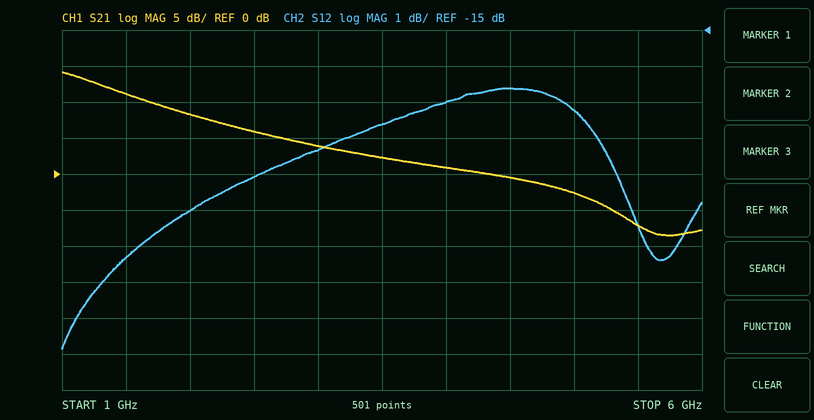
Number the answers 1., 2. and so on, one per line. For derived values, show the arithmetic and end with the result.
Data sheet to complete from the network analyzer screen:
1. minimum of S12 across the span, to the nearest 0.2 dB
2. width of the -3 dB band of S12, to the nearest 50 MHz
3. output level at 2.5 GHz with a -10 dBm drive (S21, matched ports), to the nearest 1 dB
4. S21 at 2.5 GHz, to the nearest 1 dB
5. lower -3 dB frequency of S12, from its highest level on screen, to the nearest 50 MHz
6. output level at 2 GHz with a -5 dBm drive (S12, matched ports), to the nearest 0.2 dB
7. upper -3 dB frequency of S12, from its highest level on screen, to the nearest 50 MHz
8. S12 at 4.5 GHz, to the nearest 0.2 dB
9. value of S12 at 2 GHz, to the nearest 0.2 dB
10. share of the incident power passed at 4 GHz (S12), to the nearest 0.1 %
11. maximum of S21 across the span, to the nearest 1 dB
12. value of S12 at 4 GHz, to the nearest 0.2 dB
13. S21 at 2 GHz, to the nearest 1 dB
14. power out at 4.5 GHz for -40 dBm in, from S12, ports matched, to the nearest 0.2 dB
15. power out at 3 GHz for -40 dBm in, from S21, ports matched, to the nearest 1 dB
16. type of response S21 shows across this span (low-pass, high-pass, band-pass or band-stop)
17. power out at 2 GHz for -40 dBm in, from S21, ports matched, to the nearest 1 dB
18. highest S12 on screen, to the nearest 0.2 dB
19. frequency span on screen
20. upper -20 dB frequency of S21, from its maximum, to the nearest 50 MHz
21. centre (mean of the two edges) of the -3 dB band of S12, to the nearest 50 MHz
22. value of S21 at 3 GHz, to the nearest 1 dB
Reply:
1. -23.8 dB
2. 5.40 GHz − 2.20 GHz = 3.20 GHz
3. -10 dBm + (6 dB) = -4 dBm
4. 6 dB
5. 2.20 GHz
6. -5 dBm + (-20.0 dB) = -25.0 dBm
7. 5.40 GHz
8. -16.6 dB
9. -20.0 dB
10. 10^(-17/10) ≈ 2.0 %
11. 14 dB
12. -17.0 dB
13. 8 dB
14. -40 dBm + (-16.6 dB) = -56.6 dBm
15. -40 dBm + (4 dB) = -36 dBm
16. low-pass
17. -40 dBm + (8 dB) = -32 dBm
18. -16.6 dB
19. 5 GHz
20. 5.40 GHz
21. 3.80 GHz
22. 4 dB
